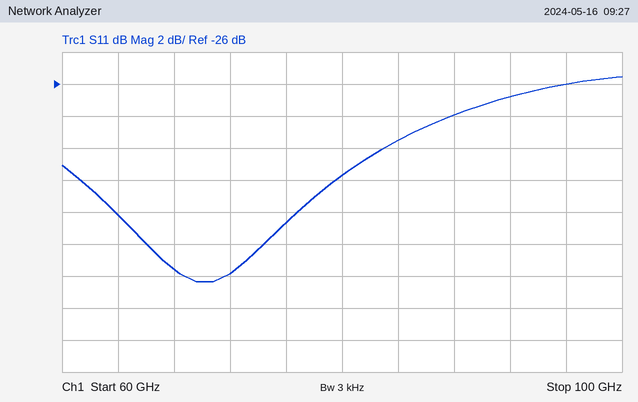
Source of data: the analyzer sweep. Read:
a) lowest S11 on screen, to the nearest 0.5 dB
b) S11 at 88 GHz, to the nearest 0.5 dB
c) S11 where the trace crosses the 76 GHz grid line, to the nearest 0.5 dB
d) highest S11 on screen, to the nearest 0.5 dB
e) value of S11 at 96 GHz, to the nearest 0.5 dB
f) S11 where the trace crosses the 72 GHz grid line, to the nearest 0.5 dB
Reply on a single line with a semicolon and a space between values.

-38.5 dB; -28.0 dB; -34.5 dB; -25.5 dB; -26.0 dB; -38.0 dB
